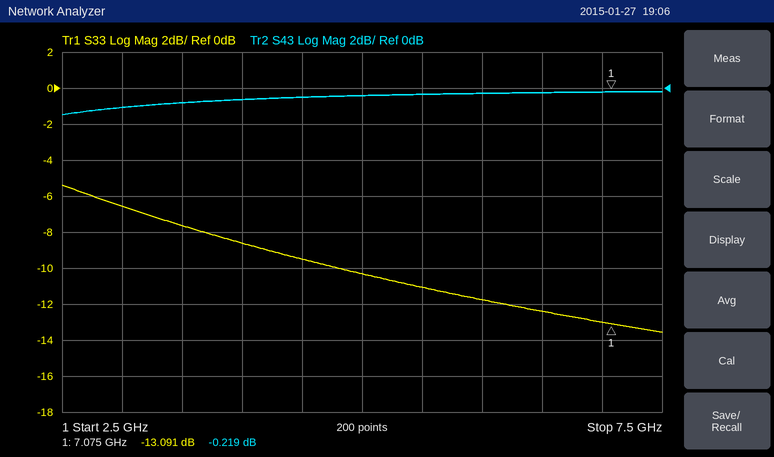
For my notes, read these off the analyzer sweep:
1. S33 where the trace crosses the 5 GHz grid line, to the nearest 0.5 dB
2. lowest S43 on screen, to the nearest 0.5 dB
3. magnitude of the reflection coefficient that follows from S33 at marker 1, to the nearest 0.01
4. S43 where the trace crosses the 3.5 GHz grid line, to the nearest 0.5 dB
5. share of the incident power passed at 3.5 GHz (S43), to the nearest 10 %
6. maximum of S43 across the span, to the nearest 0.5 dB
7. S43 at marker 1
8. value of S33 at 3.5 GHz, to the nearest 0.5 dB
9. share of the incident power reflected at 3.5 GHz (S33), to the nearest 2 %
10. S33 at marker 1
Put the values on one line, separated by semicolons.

-10.5 dB; -1.5 dB; 0.22; -1.0 dB; 80 %; 0.0 dB; -0.219 dB; -7.5 dB; 18 %; -13.091 dB
